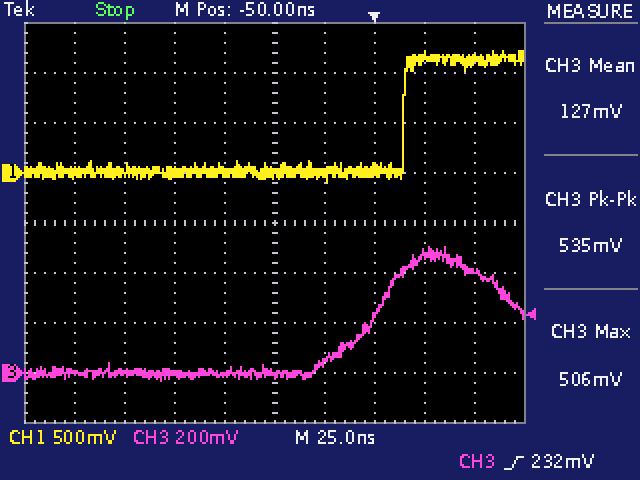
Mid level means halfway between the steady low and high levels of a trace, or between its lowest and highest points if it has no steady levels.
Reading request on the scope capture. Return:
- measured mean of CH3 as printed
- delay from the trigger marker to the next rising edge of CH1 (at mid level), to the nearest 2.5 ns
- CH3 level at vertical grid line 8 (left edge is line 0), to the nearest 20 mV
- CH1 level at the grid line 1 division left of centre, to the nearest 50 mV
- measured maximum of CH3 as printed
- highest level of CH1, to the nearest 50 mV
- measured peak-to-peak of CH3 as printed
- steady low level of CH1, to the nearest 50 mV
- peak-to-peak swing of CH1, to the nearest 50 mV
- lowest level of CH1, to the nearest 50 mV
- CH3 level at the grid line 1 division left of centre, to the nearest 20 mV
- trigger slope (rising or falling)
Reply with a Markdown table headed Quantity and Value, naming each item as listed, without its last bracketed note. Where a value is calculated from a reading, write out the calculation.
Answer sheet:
| Quantity | Value |
|---|---|
| measured mean of CH3 as printed | 127 mV |
| delay from the trigger marker to the next rising edge of CH1 (at mid level), to the nearest 2.5 ns | 15.0 ns |
| CH3 level at vertical grid line 8 (left edge is line 0), to the nearest 20 mV | 480 mV |
| CH1 level at the grid line 1 division left of centre, to the nearest 50 mV | 0 mV |
| measured maximum of CH3 as printed | 506 mV |
| highest level of CH1, to the nearest 50 mV | 1.20 V |
| measured peak-to-peak of CH3 as printed | 535 mV |
| steady low level of CH1, to the nearest 50 mV | 0 mV |
| peak-to-peak swing of CH1, to the nearest 50 mV | 1.20 V − (-100 mV) = 1.30 V |
| lowest level of CH1, to the nearest 50 mV | -100 mV |
| CH3 level at the grid line 1 division left of centre, to the nearest 20 mV | 0 mV |
| trigger slope | rising |
